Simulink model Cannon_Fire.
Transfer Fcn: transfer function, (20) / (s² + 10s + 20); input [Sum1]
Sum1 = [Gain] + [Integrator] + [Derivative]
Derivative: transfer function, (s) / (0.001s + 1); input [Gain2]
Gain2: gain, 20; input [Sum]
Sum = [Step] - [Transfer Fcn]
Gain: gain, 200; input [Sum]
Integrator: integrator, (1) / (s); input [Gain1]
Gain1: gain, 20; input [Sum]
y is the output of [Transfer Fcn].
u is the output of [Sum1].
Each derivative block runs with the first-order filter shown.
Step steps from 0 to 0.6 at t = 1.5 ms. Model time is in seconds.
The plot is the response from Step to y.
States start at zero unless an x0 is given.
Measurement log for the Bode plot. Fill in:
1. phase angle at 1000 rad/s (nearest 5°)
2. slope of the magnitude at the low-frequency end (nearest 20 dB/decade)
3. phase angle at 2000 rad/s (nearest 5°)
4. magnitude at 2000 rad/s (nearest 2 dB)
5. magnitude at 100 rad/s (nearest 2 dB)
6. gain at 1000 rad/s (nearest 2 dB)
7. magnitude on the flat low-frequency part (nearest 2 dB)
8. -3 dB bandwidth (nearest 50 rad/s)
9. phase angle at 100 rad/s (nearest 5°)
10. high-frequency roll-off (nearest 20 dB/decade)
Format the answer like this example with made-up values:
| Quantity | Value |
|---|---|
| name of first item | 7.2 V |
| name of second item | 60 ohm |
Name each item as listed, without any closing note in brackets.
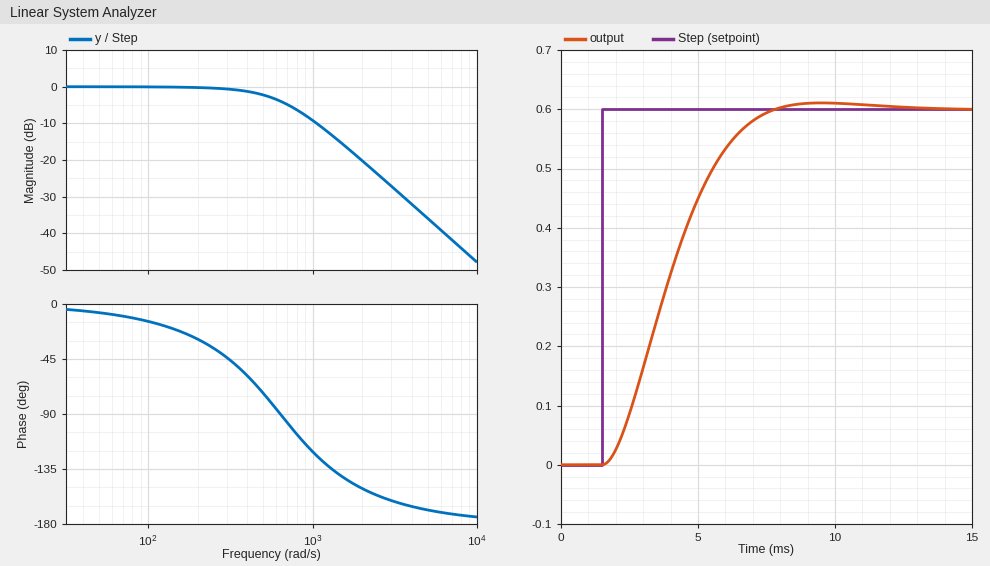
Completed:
| Quantity | Value |
|---|---|
| phase angle at 1000 rad/s | -120° |
| slope of the magnitude at the low-frequency end | 0 dB/decade |
| phase angle at 2000 rad/s | -150° |
| magnitude at 2000 rad/s | -20 dB |
| magnitude at 100 rad/s | 0 dB |
| gain at 1000 rad/s | -10 dB |
| magnitude on the flat low-frequency part | 0 dB |
| -3 dB bandwidth | 550 rad/s |
| phase angle at 100 rad/s | -15° |
| high-frequency roll-off | -40 dB/decade |
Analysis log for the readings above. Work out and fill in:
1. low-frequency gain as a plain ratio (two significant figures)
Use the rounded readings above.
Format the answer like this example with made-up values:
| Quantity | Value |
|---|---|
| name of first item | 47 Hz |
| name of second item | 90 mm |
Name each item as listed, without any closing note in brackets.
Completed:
| Quantity | Value |
|---|---|
| low-frequency gain as a plain ratio | 1.0 |
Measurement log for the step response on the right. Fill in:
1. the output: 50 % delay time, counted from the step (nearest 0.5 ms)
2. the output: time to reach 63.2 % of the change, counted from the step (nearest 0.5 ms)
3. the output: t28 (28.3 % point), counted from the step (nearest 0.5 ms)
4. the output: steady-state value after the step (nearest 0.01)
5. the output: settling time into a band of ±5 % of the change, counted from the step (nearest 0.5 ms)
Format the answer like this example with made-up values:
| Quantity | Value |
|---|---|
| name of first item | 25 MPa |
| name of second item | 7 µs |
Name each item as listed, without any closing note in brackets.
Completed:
| Quantity | Value |
|---|---|
| the output: 50 % delay time, counted from the step | 2.5 ms |
| the output: time to reach 63.2 % of the change, counted from the step | 3.0 ms |
| the output: t28 (28.3 % point), counted from the step | 1.5 ms |
| the output: steady-state value after the step | 0.60 |
| the output: settling time into a band of ±5 % of the change, counted from the step | 5.0 ms |
